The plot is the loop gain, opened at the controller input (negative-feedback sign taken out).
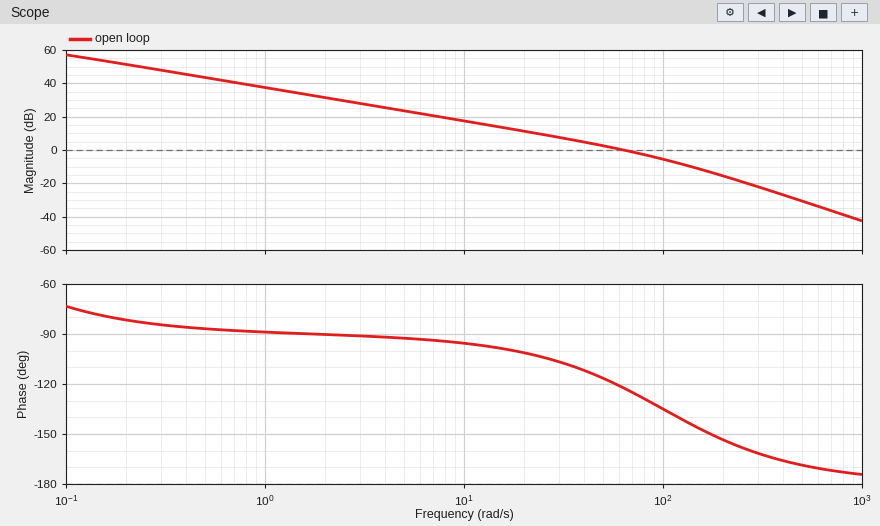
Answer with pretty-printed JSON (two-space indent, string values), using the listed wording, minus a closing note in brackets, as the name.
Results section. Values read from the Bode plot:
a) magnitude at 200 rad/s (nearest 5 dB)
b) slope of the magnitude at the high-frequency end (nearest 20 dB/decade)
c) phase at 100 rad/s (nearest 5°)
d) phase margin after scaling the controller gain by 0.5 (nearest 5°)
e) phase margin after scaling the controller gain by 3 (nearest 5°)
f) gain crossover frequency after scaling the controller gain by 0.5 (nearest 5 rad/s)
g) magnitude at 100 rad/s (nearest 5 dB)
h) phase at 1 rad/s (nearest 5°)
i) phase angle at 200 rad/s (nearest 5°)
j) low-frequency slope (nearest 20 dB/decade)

{
  "magnitude at 200 rad/s": "-15 dB",
  "slope of the magnitude at the high-frequency end": "-40 dB/decade",
  "phase at 100 rad/s": "-135°",
  "phase margin after scaling the controller gain by 0.5": "70°",
  "phase margin after scaling the controller gain by 3": "35°",
  "gain crossover frequency after scaling the controller gain by 0.5": "35 rad/s",
  "magnitude at 100 rad/s": "-5 dB",
  "phase at 1 rad/s": "-90°",
  "phase angle at 200 rad/s": "-155°",
  "low-frequency slope": "-20 dB/decade"
}
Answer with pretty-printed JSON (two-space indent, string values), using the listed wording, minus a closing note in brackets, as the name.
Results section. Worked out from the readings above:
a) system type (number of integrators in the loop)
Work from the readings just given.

{
  "system type": "1"
}
